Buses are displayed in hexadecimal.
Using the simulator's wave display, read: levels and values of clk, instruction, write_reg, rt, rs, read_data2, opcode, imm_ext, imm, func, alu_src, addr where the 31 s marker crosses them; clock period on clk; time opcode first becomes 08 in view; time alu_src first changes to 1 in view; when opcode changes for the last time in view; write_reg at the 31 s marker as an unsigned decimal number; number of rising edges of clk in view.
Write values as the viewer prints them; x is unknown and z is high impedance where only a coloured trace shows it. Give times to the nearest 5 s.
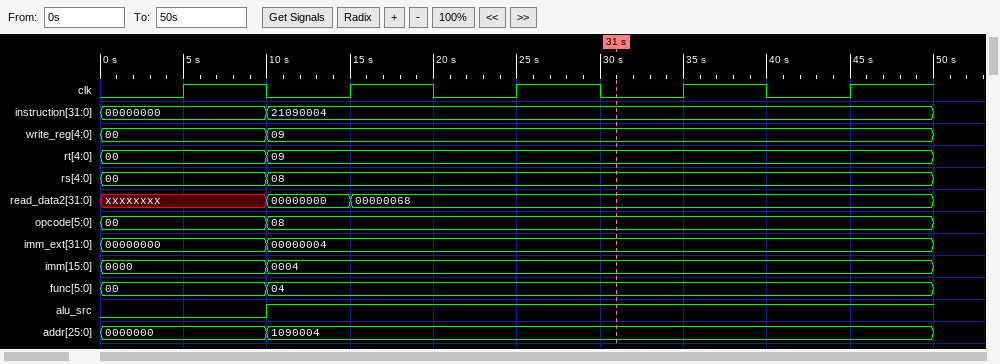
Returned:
clk=0, instruction=21090004, write_reg=09, rt=09, rs=08, read_data2=00000068, opcode=08, imm_ext=00000004, imm=0004, func=04, alu_src=1, addr=1090004
10 s
10 s
10 s
10 s
9
5
